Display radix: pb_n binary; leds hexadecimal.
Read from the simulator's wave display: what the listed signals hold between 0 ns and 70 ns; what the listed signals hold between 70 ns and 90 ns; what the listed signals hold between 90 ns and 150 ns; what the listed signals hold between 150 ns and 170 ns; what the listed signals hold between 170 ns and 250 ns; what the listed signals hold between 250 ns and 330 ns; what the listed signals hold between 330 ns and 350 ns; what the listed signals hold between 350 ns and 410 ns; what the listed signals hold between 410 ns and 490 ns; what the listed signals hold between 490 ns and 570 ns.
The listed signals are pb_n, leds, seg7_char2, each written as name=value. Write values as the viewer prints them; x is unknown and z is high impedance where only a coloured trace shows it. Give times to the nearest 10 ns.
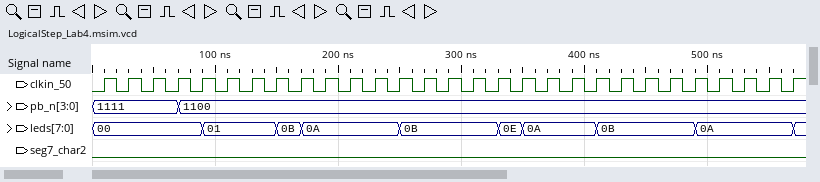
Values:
pb_n=1111, leds=00, seg7_char2=0
pb_n=1100, leds=00, seg7_char2=0
pb_n=1100, leds=01, seg7_char2=0
pb_n=1100, leds=0B, seg7_char2=0
pb_n=1100, leds=0A, seg7_char2=0
pb_n=1100, leds=0B, seg7_char2=0
pb_n=1100, leds=0E, seg7_char2=0
pb_n=1100, leds=0A, seg7_char2=0
pb_n=1100, leds=0B, seg7_char2=0
pb_n=1100, leds=0A, seg7_char2=0
